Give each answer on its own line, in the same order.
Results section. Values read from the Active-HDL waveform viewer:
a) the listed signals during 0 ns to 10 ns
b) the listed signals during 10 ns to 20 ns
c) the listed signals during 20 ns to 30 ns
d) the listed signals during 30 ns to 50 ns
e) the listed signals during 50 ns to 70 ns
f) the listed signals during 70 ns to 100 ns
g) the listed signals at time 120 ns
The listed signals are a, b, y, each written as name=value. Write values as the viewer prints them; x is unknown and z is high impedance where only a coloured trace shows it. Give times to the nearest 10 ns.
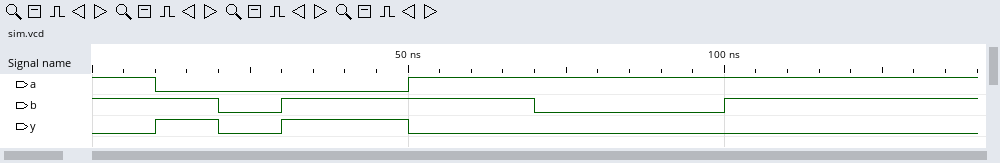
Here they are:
a=1, b=1, y=0
a=0, b=1, y=1
a=0, b=0, y=0
a=0, b=1, y=1
a=1, b=1, y=0
a=1, b=0, y=0
a=1, b=1, y=0
